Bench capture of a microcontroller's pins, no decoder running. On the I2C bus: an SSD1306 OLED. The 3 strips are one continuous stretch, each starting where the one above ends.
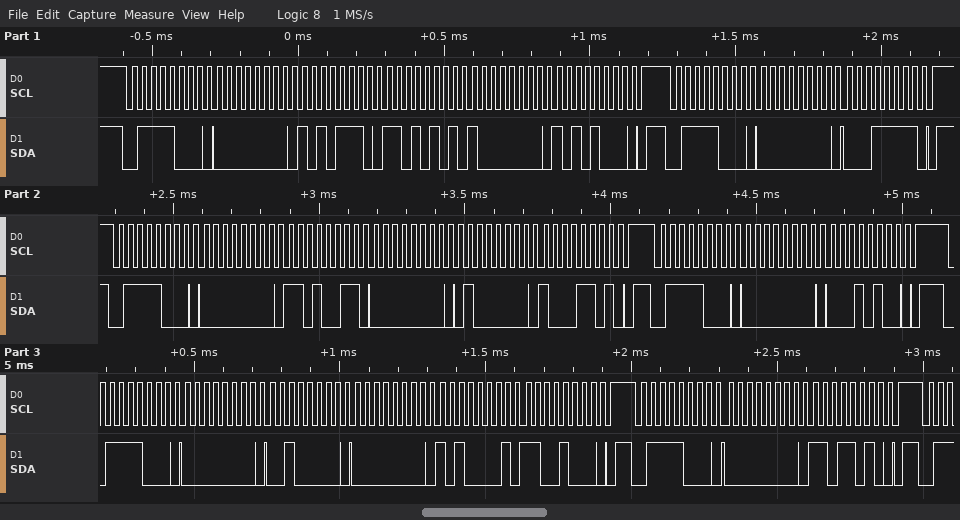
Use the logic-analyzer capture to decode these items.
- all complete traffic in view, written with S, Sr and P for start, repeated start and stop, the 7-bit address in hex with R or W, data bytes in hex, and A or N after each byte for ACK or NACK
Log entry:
S 3CW A 00 A AE A D5 A 80 A A8 A P S 3CW A 00 A 1F A P S 3CW A 00 A D3 A 00 A 40 A 8D A P S 3CW A 00 A 14 A P S 3CW A 00 A 20 A 00 A A1 A C8 A P S 3CW A 00 A DA A P
